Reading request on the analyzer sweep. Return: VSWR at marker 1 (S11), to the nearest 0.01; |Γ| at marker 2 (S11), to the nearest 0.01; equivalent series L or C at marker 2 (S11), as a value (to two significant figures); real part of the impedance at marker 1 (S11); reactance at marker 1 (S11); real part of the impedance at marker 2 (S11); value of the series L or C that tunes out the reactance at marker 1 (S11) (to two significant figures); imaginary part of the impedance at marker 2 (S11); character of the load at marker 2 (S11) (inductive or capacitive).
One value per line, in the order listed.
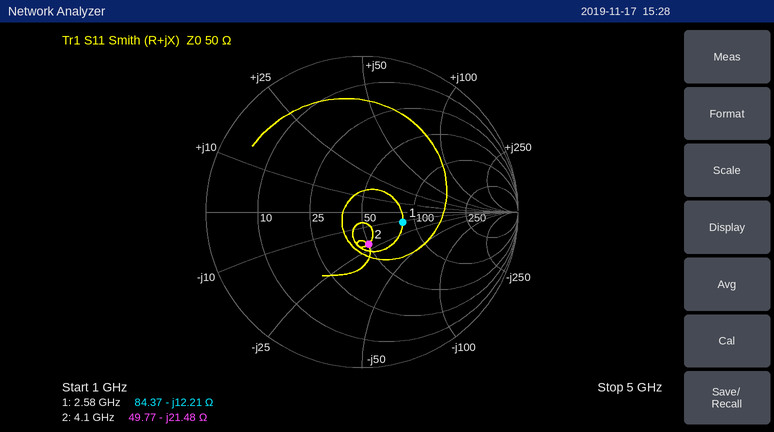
1.74
0.21
1.8 pF
84.37 Ω
-12.21 Ω
49.77 Ω
750 pH
-21.48 Ω
capacitive
